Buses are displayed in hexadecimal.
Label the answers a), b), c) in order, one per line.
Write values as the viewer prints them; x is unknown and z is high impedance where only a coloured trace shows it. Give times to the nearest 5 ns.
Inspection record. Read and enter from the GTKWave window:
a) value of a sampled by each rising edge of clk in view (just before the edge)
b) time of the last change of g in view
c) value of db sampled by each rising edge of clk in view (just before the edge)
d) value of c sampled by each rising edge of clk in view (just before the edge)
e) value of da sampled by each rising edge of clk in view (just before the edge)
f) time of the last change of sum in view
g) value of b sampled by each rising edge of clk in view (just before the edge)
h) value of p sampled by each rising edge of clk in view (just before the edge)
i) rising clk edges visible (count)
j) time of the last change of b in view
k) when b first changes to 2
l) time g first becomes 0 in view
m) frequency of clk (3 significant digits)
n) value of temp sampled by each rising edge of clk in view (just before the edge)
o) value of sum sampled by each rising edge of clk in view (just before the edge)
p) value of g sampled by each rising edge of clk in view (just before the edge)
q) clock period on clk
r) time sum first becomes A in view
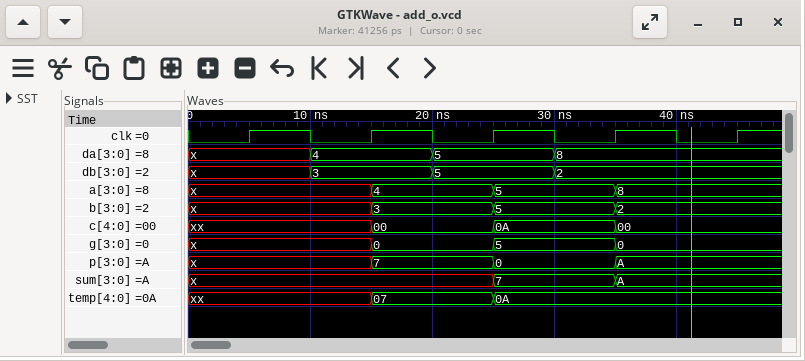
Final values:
a) x, x, 4, 5, 8
b) 35 ns
c) x, 3, 5, 2, 2
d) xx, xx, 00, 0A, 00
e) x, 4, 5, 8, 8
f) 35 ns
g) x, x, 3, 5, 2
h) x, x, 7, 0, A
i) 5
j) 35 ns
k) 35 ns
l) 15 ns
m) 100 MHz
n) xx, xx, 07, 0A, 0A
o) x, x, x, 7, A
p) x, x, 0, 5, 0
q) 10 ns
r) 35 ns
